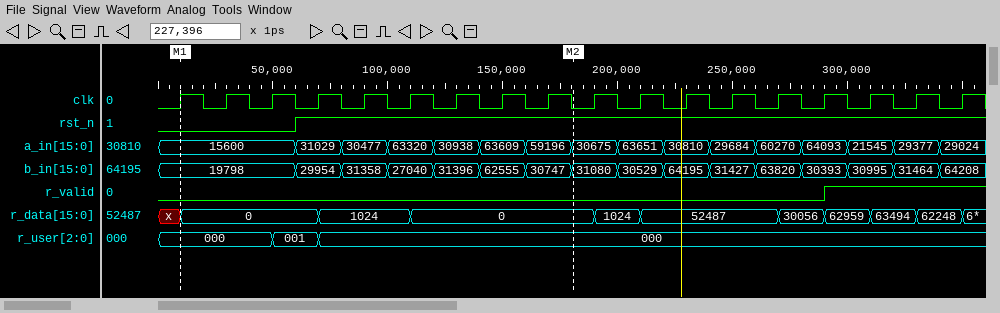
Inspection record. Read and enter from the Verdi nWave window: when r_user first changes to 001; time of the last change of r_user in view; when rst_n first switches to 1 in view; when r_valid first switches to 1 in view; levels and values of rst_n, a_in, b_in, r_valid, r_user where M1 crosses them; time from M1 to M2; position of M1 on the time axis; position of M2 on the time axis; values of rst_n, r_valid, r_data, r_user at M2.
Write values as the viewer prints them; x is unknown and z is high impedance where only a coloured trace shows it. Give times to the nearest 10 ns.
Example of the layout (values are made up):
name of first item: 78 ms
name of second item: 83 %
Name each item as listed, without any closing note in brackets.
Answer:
when r_user first changes to 001: 50 ns
time of the last change of r_user in view: 70 ns
when rst_n first switches to 1 in view: 60 ns
when r_valid first switches to 1 in view: 290 ns
levels and values of rst_n, a_in, b_in, r_valid, r_user where M1 crosses them: rst_n=0, a_in=15600, b_in=19798, r_valid=0, r_user=000
time from M1 to M2: 170 ns
position of M1 on the time axis: 10 ns
position of M2 on the time axis: 180 ns
values of rst_n, r_valid, r_data, r_user at M2: rst_n=1, r_valid=0, r_data=0, r_user=000
